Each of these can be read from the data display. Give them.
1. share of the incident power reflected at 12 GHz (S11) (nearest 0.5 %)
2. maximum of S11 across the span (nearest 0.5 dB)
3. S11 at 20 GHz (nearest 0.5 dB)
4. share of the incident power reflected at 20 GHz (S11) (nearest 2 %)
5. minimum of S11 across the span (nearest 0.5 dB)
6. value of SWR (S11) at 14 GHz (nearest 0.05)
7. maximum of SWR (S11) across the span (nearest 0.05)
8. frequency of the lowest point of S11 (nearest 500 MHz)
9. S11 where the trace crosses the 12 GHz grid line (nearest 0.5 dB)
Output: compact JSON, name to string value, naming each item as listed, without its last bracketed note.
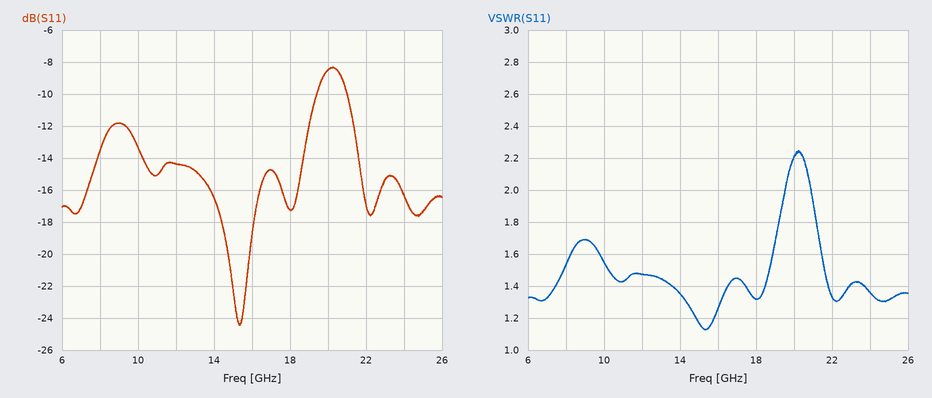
{"share of the incident power reflected at 12 GHz (S11)": "3.5 %", "maximum of S11 across the span": "-8.5 dB", "S11 at 20 GHz": "-8.5 dB", "share of the incident power reflected at 20 GHz (S11)": "14 %", "minimum of S11 across the span": "-24.5 dB", "value of SWR (S11) at 14 GHz": "1.35", "maximum of SWR (S11) across the span": "2.25", "frequency of the lowest point of S11": "15.5 GHz", "S11 where the trace crosses the 12 GHz grid line": "-14.5 dB"}
